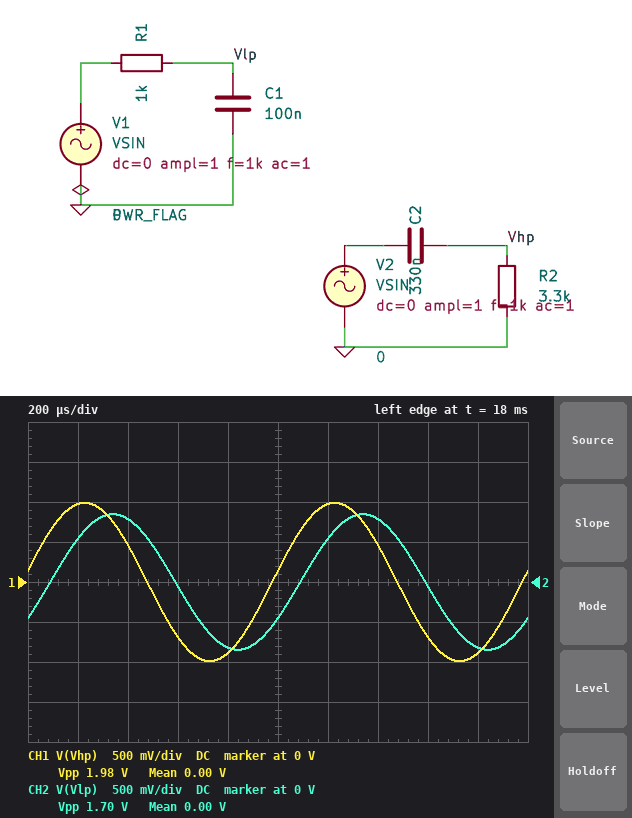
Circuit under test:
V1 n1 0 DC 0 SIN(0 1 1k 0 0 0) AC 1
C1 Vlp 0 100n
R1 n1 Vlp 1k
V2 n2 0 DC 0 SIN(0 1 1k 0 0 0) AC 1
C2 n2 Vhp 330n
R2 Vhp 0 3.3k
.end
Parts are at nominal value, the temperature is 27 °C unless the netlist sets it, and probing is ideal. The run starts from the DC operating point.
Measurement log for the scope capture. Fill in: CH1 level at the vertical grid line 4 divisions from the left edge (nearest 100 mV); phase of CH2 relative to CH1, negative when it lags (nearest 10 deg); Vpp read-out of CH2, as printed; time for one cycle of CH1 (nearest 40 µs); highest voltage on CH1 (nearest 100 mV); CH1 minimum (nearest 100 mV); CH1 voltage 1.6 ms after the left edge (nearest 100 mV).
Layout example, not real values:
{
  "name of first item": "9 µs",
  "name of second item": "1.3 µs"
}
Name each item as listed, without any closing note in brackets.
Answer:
{
  "CH1 level at the vertical grid line 4 divisions from the left edge": "-900 mV",
  "phase of CH2 relative to CH1, negative when it lags": "-40 deg",
  "Vpp read-out of CH2, as printed": "1.70 V",
  "time for one cycle of CH1": "1.00 ms",
  "highest voltage on CH1": "1.0 V",
  "CH1 minimum": "-1.0 V",
  "CH1 voltage 1.6 ms after the left edge": "-700 mV"
}
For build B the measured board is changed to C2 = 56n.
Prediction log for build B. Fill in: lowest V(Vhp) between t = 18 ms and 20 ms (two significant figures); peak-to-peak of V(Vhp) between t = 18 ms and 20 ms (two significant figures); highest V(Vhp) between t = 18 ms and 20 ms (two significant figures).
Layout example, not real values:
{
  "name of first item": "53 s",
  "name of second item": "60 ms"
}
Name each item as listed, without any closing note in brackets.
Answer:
{
  "lowest V(Vhp) between t = 18 ms and 20 ms": "-760 mV",
  "peak-to-peak of V(Vhp) between t = 18 ms and 20 ms": "1.5 V",
  "highest V(Vhp) between t = 18 ms and 20 ms": "760 mV"
}
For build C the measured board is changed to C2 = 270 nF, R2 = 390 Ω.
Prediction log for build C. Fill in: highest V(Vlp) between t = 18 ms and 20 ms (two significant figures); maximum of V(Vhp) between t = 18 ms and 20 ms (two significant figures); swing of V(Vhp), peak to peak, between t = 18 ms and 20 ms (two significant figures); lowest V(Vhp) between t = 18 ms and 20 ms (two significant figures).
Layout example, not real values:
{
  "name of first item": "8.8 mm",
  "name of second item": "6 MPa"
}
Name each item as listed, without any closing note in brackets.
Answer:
{
  "highest V(Vlp) between t = 18 ms and 20 ms": "850 mV",
  "maximum of V(Vhp) between t = 18 ms and 20 ms": "550 mV",
  "swing of V(Vhp), peak to peak, between t = 18 ms and 20 ms": "1.1 V",
  "lowest V(Vhp) between t = 18 ms and 20 ms": "-550 mV"
}
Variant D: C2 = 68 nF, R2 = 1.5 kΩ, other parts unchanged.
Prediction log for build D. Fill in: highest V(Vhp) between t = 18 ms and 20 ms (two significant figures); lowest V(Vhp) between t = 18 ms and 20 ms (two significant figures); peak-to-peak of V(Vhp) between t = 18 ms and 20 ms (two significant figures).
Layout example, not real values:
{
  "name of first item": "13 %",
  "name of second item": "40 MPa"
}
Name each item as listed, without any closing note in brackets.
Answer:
{
  "highest V(Vhp) between t = 18 ms and 20 ms": "540 mV",
  "lowest V(Vhp) between t = 18 ms and 20 ms": "-540 mV",
  "peak-to-peak of V(Vhp) between t = 18 ms and 20 ms": "1.1 V"
}
